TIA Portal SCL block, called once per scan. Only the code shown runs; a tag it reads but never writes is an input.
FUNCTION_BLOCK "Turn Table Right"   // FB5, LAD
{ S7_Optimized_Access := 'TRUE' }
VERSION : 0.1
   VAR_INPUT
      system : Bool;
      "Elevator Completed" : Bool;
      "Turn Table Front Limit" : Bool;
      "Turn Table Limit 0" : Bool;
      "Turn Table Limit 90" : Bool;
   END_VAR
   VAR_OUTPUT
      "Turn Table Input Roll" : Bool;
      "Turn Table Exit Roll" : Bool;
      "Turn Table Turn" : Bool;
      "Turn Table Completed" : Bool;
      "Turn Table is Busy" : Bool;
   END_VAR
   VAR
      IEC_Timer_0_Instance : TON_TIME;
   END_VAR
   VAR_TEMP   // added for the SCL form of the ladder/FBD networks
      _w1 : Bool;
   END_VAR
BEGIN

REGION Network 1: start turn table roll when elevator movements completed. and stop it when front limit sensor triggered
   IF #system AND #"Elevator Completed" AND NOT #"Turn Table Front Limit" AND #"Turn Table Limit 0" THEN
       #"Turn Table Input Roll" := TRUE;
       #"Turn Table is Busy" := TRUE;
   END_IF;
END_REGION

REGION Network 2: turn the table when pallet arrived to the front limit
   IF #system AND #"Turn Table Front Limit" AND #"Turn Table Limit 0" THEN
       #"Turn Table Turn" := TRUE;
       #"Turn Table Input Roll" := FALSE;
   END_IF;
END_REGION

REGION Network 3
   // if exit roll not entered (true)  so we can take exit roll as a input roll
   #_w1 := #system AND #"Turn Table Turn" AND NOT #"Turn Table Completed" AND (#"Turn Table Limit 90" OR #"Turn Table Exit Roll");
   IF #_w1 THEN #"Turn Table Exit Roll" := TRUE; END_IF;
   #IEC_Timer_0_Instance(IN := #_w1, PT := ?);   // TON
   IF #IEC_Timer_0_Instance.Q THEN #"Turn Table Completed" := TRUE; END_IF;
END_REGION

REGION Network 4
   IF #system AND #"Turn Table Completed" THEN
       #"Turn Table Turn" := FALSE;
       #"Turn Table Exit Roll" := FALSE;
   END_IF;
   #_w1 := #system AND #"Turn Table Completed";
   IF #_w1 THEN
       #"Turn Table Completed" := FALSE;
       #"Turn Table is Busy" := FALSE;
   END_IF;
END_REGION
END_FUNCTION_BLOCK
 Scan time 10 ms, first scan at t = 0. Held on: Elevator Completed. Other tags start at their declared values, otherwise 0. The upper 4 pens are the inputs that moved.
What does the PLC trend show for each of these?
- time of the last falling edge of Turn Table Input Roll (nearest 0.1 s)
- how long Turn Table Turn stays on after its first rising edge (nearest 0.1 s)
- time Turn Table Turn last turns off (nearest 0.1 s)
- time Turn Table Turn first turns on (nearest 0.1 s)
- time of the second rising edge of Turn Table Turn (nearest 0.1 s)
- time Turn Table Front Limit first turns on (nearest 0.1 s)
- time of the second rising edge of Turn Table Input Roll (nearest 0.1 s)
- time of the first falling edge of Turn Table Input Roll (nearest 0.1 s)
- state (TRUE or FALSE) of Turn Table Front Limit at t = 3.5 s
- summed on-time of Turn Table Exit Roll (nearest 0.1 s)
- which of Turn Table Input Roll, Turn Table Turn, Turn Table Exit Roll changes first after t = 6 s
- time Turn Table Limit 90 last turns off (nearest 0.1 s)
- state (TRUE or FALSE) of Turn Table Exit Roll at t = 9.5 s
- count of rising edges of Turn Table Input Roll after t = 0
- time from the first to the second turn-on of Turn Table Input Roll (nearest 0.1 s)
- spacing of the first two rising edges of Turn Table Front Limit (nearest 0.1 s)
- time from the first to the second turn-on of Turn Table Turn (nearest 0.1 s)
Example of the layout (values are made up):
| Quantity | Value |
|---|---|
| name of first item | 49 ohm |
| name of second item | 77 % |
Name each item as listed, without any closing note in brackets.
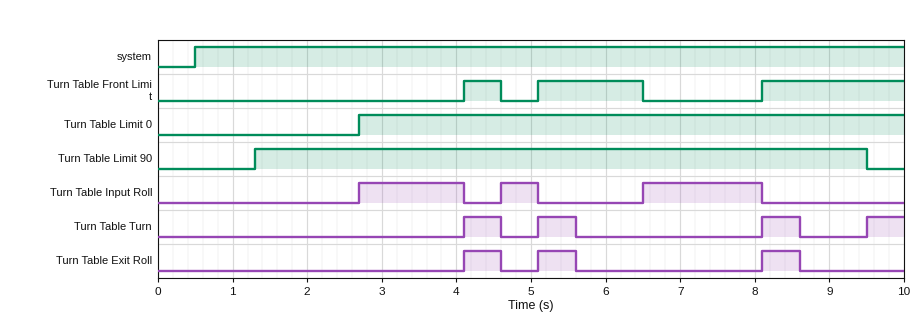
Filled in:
| Quantity | Value |
|---|---|
| time of the last falling edge of Turn Table Input Roll | 8.1 s |
| how long Turn Table Turn stays on after its first rising edge | 0.5 s |
| time Turn Table Turn last turns off | 8.6 s |
| time Turn Table Turn first turns on | 4.1 s |
| time of the second rising edge of Turn Table Turn | 5.1 s |
| time Turn Table Front Limit first turns on | 4.1 s |
| time of the second rising edge of Turn Table Input Roll | 4.6 s |
| time of the first falling edge of Turn Table Input Roll | 4.1 s |
| state (TRUE or FALSE) of Turn Table Front Limit at t = 3.5 s | FALSE |
| summed on-time of Turn Table Exit Roll | 1.5 s |
| which of Turn Table Input Roll, Turn Table Turn, Turn Table Exit Roll changes first after t = 6 s | Turn Table Input Roll |
| time Turn Table Limit 90 last turns off | 9.5 s |
| state (TRUE or FALSE) of Turn Table Exit Roll at t = 9.5 s | FALSE |
| count of rising edges of Turn Table Input Roll after t = 0 | 3 |
| time from the first to the second turn-on of Turn Table Input Roll | 1.9 s |
| spacing of the first two rising edges of Turn Table Front Limit | 1.0 s |
| time from the first to the second turn-on of Turn Table Turn | 1.0 s |
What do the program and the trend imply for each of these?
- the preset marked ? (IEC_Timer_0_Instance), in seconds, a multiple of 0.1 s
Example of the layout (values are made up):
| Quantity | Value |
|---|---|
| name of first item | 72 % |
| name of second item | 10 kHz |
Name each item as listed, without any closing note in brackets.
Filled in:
| Quantity | Value |
|---|---|
| the preset marked ? (IEC_Timer_0_Instance), in seconds, a multiple of 0.1 s | 0.5 s |
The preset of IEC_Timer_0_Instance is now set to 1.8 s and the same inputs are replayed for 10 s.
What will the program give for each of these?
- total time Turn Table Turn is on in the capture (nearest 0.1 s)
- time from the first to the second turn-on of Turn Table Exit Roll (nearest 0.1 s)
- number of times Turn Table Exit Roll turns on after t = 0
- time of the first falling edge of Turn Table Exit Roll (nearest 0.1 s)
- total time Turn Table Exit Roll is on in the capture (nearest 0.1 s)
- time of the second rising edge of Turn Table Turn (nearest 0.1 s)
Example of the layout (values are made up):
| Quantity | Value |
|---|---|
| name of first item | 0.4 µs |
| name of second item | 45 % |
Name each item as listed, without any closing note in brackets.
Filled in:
| Quantity | Value |
|---|---|
| total time Turn Table Turn is on in the capture | 3.7 s |
| time from the first to the second turn-on of Turn Table Exit Roll | 4.0 s |
| number of times Turn Table Exit Roll turns on after t = 0 | 2 |
| time of the first falling edge of Turn Table Exit Roll | 5.9 s |
| total time Turn Table Exit Roll is on in the capture | 3.6 s |
| time of the second rising edge of Turn Table Turn | 8.1 s |
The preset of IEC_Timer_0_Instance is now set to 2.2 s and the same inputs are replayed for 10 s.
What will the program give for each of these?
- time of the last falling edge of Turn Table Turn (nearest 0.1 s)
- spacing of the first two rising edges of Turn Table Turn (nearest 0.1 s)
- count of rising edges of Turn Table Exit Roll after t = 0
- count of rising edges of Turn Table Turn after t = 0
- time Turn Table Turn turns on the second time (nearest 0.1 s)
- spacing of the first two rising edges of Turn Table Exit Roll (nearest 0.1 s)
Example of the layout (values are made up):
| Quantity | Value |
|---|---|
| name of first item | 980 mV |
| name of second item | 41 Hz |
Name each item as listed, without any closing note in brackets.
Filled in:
| Quantity | Value |
|---|---|
| time of the last falling edge of Turn Table Turn | 6.3 s |
| spacing of the first two rising edges of Turn Table Turn | 4.0 s |
| count of rising edges of Turn Table Exit Roll after t = 0 | 2 |
| count of rising edges of Turn Table Turn after t = 0 | 2 |
| time Turn Table Turn turns on the second time | 8.1 s |
| spacing of the first two rising edges of Turn Table Exit Roll | 4.0 s |
